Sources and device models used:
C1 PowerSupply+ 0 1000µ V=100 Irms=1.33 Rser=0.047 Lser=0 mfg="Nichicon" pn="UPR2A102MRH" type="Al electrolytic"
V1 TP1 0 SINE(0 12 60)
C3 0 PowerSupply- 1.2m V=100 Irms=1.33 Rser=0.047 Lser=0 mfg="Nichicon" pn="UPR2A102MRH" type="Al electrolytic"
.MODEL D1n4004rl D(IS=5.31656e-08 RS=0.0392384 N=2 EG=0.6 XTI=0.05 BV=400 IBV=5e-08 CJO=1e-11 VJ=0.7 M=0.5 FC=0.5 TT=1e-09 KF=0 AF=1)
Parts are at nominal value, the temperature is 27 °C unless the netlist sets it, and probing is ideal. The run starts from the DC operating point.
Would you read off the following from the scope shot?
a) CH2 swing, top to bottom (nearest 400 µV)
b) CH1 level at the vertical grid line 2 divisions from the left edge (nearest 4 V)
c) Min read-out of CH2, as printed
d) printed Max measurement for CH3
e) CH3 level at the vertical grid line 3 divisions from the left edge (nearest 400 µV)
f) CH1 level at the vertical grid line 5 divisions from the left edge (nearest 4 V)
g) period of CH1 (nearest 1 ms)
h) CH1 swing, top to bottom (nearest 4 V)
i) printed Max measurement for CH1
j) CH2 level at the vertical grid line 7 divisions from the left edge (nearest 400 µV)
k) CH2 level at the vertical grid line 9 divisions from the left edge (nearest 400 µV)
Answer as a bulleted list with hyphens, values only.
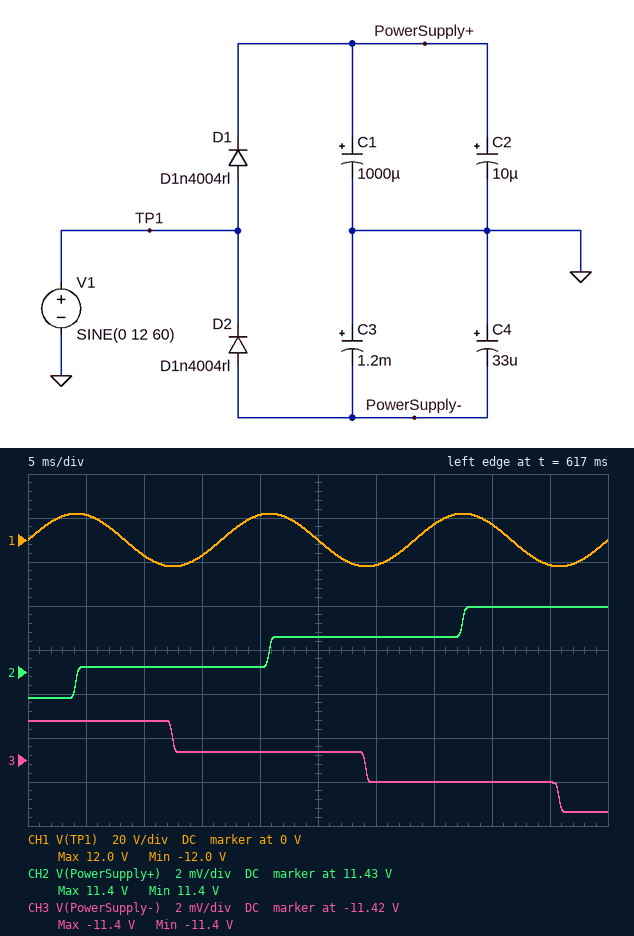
- 4.0 mV
- -8 V
- 11.4 V
- -11.4 V
- -11.4196 V
- 0 V
- 17 ms
- 24 V
- 12.0 V
- 11.4316 V
- 11.4328 V
